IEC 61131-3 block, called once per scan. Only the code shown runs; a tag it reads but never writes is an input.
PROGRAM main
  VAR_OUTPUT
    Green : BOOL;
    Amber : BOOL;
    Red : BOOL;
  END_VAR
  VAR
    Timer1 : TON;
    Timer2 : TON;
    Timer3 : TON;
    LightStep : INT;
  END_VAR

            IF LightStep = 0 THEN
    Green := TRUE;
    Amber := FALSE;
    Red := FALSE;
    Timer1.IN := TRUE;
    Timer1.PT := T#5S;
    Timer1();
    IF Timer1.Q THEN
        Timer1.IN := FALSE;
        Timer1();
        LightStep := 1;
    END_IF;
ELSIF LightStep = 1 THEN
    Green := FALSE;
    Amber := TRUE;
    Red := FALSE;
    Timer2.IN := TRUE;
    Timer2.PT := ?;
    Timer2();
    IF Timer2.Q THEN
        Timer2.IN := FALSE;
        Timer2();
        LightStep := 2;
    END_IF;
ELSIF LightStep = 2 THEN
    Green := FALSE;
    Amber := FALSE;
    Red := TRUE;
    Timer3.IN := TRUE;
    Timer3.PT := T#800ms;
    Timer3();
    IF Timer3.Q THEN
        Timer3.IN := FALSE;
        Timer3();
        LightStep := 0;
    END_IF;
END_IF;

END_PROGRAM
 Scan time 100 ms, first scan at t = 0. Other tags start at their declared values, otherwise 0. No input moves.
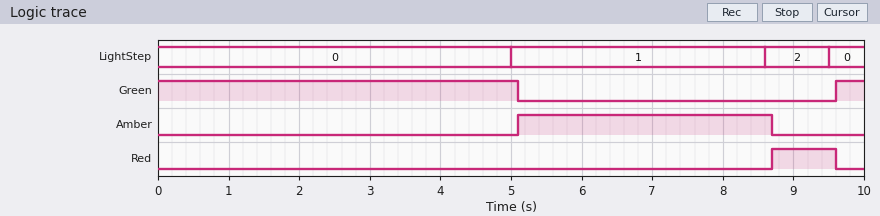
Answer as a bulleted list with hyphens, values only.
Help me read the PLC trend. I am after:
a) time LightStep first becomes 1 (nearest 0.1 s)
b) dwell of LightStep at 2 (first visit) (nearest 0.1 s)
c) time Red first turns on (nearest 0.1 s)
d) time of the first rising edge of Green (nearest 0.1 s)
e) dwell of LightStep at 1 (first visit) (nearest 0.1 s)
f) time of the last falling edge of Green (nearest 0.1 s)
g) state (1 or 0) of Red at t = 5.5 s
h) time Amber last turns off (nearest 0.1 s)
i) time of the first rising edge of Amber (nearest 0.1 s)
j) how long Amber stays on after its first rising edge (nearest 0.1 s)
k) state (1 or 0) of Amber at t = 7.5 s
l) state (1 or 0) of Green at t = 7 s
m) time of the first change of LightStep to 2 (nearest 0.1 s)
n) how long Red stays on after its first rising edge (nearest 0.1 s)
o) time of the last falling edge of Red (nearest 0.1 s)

- 5.0 s
- 0.9 s
- 8.7 s
- 9.6 s
- 3.6 s
- 5.1 s
- 0
- 8.7 s
- 5.1 s
- 3.6 s
- 1
- 0
- 8.6 s
- 0.9 s
- 9.6 s
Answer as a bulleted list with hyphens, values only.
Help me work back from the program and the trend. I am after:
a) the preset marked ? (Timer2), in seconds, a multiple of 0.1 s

- 3.5 s
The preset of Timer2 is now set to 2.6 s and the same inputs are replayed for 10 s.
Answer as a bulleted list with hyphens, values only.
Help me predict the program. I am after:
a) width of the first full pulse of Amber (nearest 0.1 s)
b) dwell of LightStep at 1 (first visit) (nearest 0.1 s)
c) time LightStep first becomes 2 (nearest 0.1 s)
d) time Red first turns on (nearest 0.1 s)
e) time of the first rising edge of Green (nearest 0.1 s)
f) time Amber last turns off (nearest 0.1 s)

- 2.7 s
- 2.7 s
- 7.7 s
- 7.8 s
- 8.7 s
- 7.8 s
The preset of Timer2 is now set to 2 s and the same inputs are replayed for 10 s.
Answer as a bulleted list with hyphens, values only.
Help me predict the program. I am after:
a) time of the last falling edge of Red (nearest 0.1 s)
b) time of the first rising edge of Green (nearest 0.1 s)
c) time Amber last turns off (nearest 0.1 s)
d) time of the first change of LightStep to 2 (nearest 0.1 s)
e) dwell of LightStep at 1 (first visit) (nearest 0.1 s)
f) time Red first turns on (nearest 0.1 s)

- 8.1 s
- 8.1 s
- 7.2 s
- 7.1 s
- 2.1 s
- 7.2 s
